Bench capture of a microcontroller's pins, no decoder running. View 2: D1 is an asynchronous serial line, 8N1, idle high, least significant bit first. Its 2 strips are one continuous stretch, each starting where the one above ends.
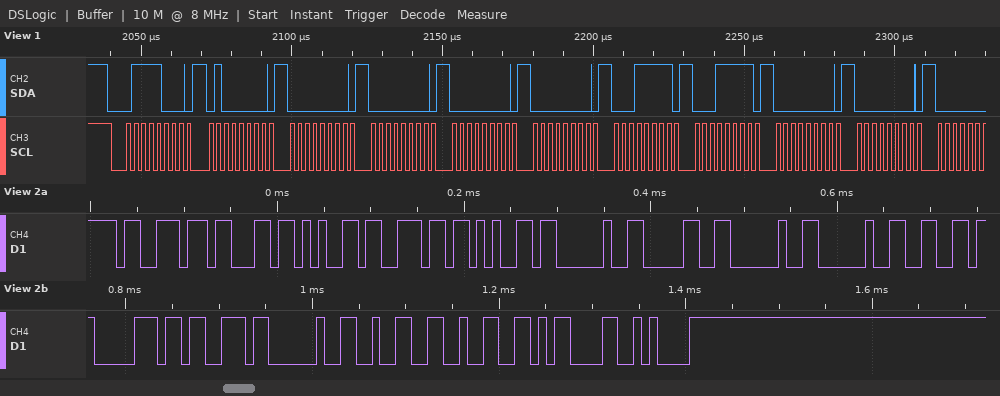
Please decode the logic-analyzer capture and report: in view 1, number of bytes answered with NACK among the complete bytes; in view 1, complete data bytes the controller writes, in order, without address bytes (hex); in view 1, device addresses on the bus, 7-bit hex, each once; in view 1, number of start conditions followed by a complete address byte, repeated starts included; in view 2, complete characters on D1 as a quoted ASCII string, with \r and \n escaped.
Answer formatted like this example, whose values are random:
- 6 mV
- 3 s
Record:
- 0
- 40 00 00 00 00 1F 1F 00 00
- 0x3C
- 1
- "scene 0  fps 22\r\n"
